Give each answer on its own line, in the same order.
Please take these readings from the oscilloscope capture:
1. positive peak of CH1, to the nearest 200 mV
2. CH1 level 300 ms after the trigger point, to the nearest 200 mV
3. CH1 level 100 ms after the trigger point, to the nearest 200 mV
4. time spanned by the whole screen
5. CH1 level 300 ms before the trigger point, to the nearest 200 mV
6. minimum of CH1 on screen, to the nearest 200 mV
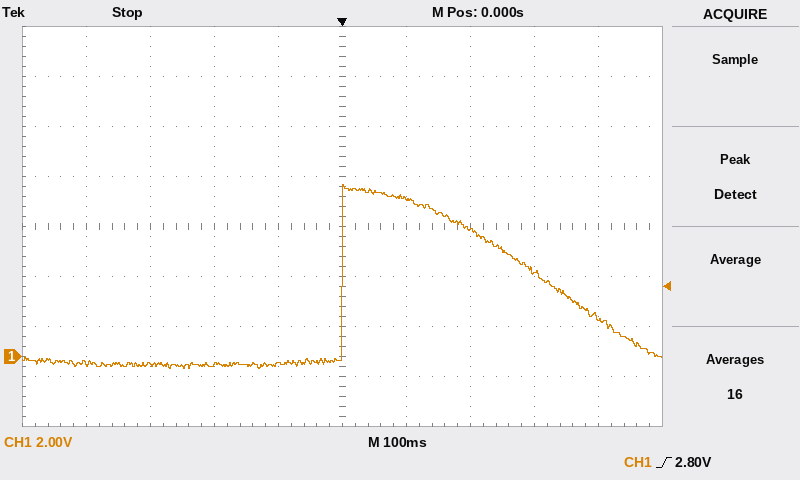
6.8 V
3.4 V
6.4 V
1 s
-400 mV
-400 mV
